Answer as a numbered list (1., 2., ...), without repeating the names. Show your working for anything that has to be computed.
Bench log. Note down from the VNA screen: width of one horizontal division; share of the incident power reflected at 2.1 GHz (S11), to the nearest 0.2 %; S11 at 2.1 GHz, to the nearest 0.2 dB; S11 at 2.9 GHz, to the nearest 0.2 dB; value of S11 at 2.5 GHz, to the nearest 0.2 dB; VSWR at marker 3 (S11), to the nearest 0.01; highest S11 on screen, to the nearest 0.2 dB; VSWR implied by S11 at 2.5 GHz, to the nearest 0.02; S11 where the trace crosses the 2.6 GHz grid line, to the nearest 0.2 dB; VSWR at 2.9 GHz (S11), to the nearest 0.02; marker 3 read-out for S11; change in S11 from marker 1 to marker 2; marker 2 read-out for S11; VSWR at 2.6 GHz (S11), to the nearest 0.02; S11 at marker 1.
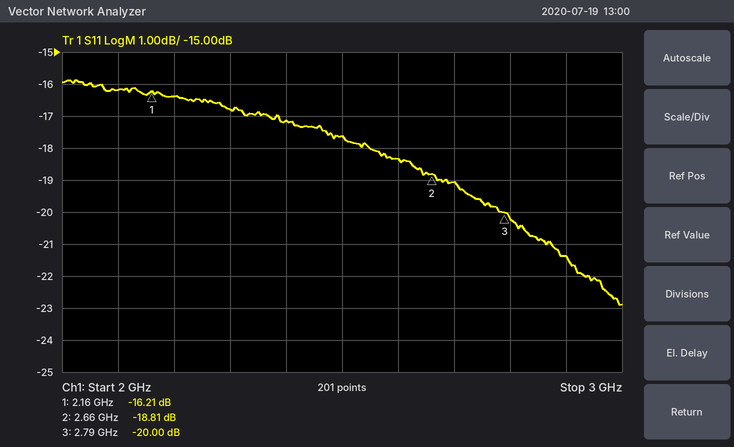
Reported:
1. 100 MHz
2. 10^(-16.2/10) ≈ 2.4 %
3. -16.2 dB
4. -21.4 dB
5. -17.6 dB
6. (1 + 0.1000)/(1 − 0.1000) ≈ 1.22
7. -15.8 dB
8. |Γ| = 10^(-17.6/20) = 0.1318; VSWR = (1 + 0.1318)/(1 − 0.1318) ≈ 1.30
9. -18.4 dB
10. |Γ| = 10^(-21.4/20) = 0.0851; VSWR = (1 + 0.0851)/(1 − 0.0851) ≈ 1.19, so 1.18 to the nearest 0.02
11. -20.00 dB
12. -18.81 − (-16.21) = -2.60 dB
13. -18.81 dB
14. |Γ| = 10^(-18.4/20) = 0.1202; VSWR = (1 + 0.1202)/(1 − 0.1202) ≈ 1.27, so 1.28 to the nearest 0.02
15. -16.21 dB
